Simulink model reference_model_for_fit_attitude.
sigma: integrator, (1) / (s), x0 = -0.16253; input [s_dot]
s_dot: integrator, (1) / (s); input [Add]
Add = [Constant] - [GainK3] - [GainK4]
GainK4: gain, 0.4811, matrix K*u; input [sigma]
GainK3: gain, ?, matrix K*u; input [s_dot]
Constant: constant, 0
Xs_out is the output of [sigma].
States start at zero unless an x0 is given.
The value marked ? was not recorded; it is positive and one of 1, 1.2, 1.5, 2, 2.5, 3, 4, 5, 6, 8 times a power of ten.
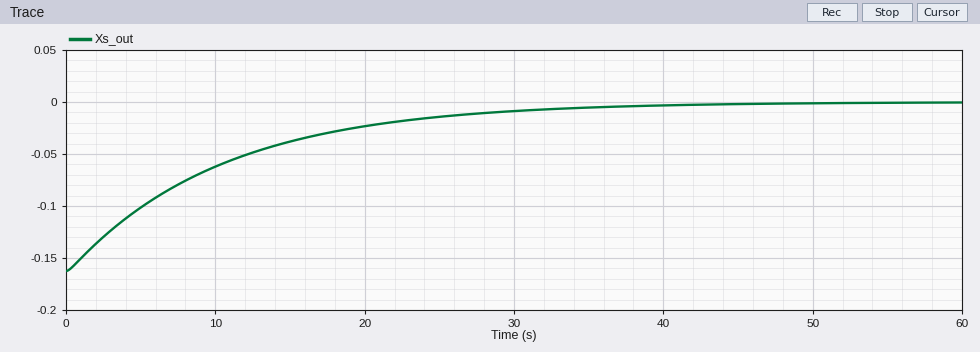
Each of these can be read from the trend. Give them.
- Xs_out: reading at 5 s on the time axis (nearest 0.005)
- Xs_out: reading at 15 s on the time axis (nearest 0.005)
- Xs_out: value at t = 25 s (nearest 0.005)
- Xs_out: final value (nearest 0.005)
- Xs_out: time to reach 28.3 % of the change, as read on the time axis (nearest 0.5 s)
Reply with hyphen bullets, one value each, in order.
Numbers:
- -0.100
- -0.040
- -0.015
- 0.000
- 3.5 s
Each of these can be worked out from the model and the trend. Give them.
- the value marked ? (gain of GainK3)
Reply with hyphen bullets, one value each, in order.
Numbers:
- 5
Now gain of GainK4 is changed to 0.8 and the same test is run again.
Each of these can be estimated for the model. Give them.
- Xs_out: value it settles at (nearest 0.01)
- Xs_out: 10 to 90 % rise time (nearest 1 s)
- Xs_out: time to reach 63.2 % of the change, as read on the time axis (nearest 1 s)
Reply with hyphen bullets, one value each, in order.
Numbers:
- 0.00
- 13 s
- 6 s
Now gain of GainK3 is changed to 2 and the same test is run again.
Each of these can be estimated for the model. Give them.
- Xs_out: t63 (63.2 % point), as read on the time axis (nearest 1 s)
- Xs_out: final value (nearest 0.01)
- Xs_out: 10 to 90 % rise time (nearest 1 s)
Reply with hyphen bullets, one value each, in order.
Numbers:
- 4 s
- 0.00
- 8 s
